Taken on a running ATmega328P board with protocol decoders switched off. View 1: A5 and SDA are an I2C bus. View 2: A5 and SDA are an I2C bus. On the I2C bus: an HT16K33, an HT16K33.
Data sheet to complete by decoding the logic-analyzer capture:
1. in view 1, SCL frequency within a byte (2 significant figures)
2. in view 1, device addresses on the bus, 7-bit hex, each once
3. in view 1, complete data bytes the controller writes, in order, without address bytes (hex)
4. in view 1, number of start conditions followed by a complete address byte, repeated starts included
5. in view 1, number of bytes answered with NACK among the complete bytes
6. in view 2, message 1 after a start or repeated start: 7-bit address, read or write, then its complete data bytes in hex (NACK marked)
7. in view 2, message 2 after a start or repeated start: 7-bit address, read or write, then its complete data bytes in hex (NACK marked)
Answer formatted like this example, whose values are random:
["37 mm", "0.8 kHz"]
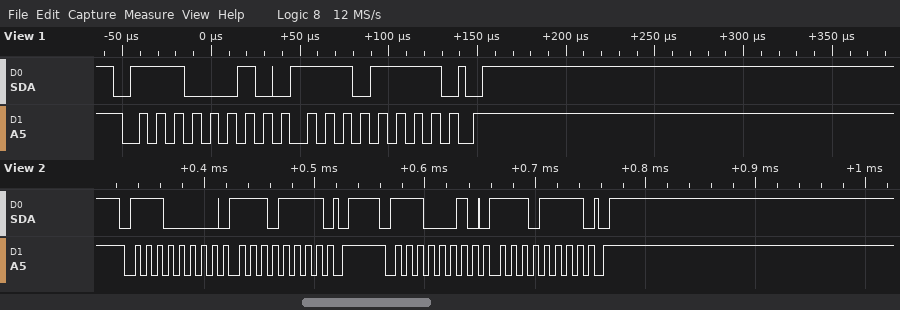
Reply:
["100 kHz", "0x71", "EF", "1", "0", "0x70 write: EF", "0x71 write: EF"]
